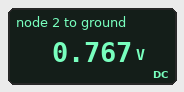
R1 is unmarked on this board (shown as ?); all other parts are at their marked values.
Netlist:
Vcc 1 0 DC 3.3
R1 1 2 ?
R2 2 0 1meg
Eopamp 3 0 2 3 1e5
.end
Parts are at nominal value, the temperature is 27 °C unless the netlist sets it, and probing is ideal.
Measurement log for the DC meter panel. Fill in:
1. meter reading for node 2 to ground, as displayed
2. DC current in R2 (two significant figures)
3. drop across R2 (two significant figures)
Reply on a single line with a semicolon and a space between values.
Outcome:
0.767 V; 770 nA; 770 mV
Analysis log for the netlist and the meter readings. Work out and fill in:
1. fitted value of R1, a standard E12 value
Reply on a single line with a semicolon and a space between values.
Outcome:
3.3 MΩ
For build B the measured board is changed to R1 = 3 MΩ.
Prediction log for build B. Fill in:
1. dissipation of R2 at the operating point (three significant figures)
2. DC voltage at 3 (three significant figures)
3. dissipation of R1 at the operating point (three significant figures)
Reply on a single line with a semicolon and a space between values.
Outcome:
681 nW; 825 mV; 2.04 µW
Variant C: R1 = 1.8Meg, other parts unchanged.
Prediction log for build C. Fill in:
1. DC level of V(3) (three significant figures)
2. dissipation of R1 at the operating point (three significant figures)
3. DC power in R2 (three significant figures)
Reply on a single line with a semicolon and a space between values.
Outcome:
1.18 V; 2.50 µW; 1.39 µW
